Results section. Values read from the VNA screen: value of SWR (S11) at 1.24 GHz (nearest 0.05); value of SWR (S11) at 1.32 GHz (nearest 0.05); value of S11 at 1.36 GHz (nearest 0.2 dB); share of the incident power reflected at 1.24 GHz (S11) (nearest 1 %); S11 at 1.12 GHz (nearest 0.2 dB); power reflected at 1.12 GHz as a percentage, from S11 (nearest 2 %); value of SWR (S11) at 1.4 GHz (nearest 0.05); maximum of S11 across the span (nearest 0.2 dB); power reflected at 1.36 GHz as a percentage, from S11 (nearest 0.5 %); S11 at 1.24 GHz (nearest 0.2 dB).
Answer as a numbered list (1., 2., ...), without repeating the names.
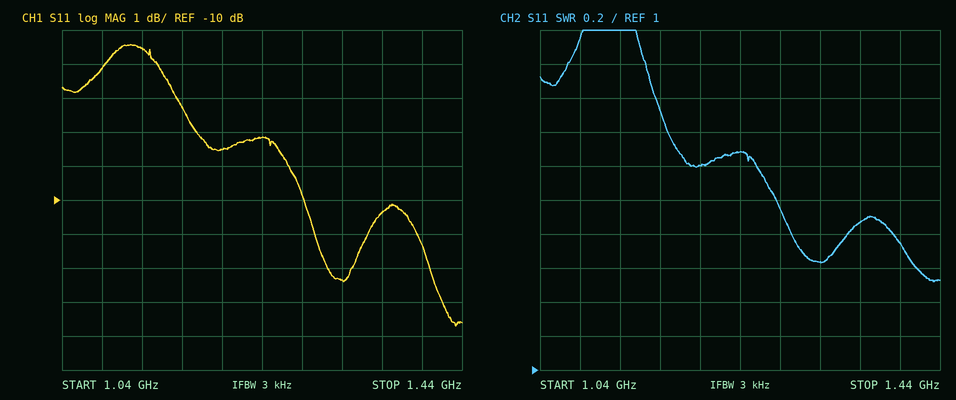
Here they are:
1. 2.30
2. 1.65
3. -10.4 dB
4. 15 %
5. -5.6 dB
6. 28 %
7. 1.75
8. -5.4 dB
9. 9.0 %
10. -8.2 dB
